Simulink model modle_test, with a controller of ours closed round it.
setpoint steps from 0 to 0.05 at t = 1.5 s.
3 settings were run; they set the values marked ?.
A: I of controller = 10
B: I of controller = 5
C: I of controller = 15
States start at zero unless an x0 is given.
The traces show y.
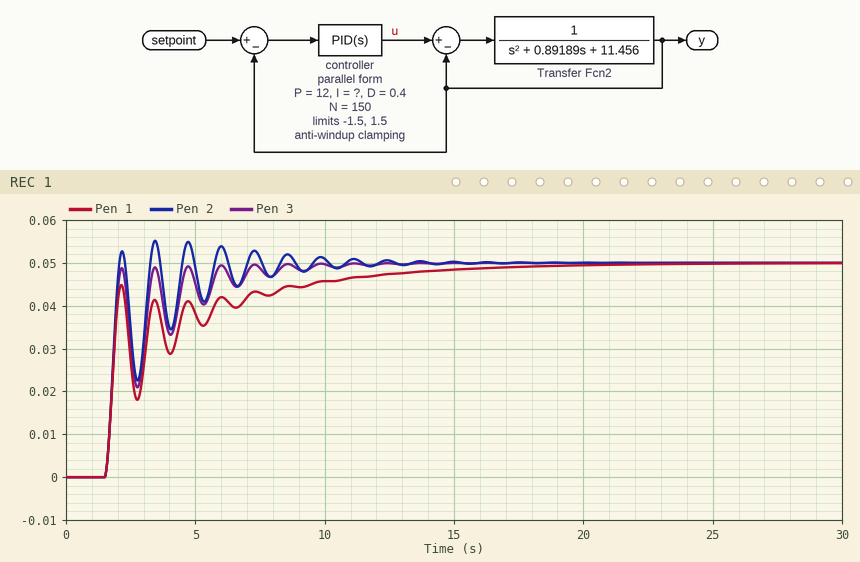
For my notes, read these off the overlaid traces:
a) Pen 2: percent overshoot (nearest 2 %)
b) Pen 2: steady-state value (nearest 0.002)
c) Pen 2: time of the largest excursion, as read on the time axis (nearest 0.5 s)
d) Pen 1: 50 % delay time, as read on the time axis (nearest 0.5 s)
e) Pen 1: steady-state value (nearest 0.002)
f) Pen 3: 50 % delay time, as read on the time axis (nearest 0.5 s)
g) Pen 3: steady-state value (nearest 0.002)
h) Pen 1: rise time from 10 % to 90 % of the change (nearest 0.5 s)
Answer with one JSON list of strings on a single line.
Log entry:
["10 %", "0.050", "3.5 s", "2.0 s", "0.050", "2.0 s", "0.050", "8.0 s"]
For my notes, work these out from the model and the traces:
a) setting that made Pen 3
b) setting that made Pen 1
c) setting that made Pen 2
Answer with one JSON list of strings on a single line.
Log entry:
["A", "B", "C"]
